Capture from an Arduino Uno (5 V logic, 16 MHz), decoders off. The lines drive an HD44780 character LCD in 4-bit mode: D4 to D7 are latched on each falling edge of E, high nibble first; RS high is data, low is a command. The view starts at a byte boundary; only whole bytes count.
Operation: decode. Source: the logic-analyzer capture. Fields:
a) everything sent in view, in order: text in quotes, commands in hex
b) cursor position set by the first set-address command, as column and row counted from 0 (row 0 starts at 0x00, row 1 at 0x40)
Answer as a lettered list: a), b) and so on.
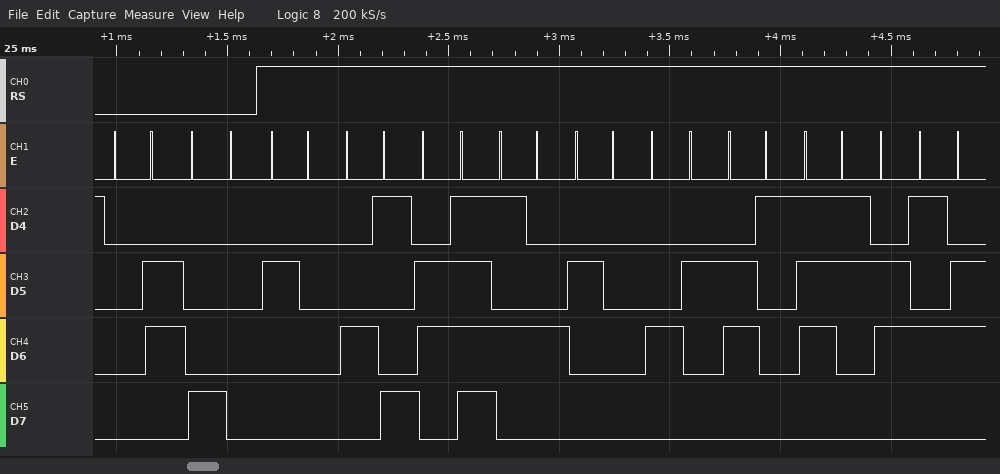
a) 0x06 0x80 " IoT Base"
b) column 0, row 0
